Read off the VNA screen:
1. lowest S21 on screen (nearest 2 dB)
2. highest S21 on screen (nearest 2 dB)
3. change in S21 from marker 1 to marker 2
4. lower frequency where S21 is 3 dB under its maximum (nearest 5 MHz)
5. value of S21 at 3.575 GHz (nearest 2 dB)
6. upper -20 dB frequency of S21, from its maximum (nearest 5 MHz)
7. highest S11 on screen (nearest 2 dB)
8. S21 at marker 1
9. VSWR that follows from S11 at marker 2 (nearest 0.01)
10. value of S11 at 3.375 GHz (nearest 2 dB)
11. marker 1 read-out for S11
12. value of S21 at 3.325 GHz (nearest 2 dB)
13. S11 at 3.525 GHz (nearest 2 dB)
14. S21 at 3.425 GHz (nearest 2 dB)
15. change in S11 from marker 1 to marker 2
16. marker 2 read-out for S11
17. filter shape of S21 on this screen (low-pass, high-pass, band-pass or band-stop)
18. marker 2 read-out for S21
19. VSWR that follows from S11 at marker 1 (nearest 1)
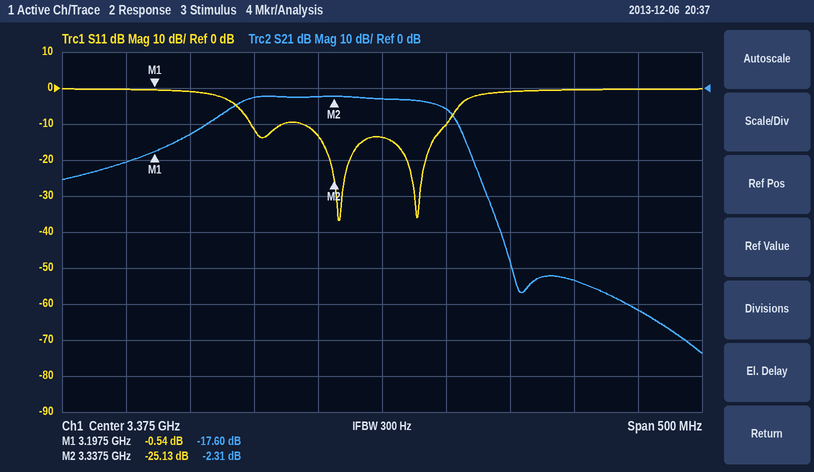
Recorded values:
-74 dB
-2 dB
15.29 dB
3.260 GHz
-62 dB
3.450 GHz
0 dB
-17.60 dB
1.12
-14 dB
-0.54 dB
-2 dB
0 dB
-6 dB
-24.59 dB
-25.13 dB
band-pass
-2.31 dB
32
